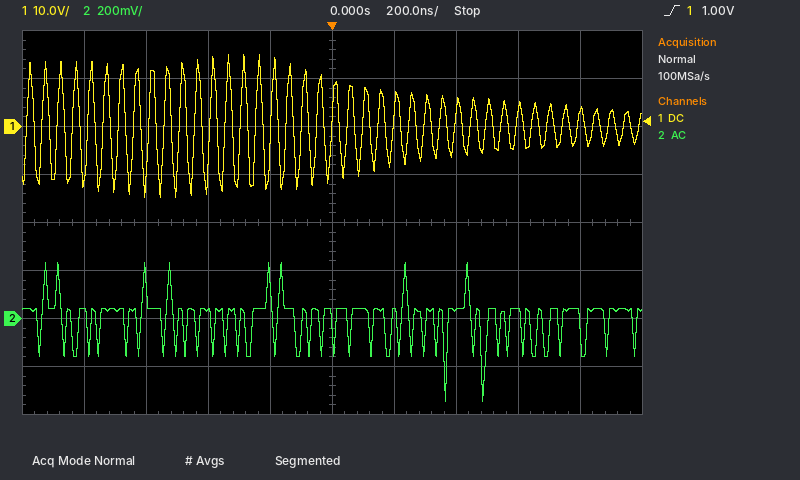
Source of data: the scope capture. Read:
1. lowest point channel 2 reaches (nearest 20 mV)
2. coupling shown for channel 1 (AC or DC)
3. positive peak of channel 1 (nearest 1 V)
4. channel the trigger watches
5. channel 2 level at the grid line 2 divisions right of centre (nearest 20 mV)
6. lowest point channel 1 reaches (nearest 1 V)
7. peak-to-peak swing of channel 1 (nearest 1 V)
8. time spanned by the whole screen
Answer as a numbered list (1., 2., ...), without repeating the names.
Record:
1. -340 mV
2. DC
3. 15 V
4. channel 1
5. 40 mV
6. -15 V
7. 30 V
8. 2 µs
